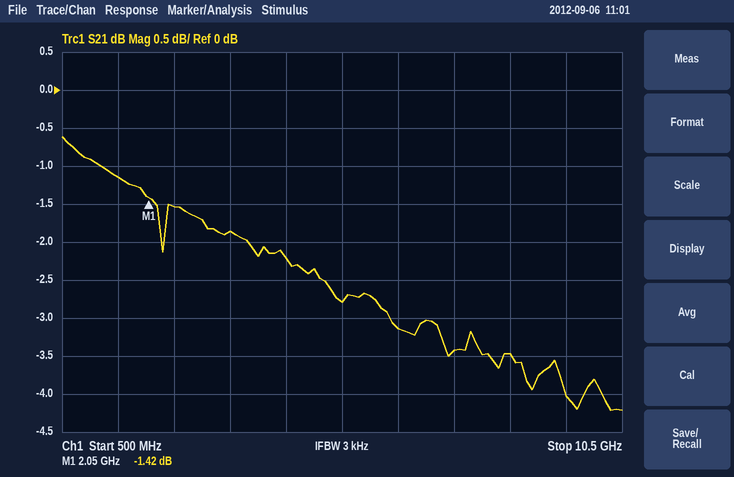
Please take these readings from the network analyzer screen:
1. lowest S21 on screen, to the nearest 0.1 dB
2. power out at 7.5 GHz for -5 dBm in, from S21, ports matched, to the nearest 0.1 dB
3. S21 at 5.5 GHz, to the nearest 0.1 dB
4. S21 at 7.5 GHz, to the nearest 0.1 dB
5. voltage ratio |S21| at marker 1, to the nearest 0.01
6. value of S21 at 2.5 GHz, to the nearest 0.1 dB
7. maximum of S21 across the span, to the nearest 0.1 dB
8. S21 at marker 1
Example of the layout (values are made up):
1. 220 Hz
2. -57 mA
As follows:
1. -4.2 dB
2. -8.4 dBm
3. -2.8 dB
4. -3.4 dB
5. 0.85
6. -1.5 dB
7. -0.6 dB
8. -1.42 dB
